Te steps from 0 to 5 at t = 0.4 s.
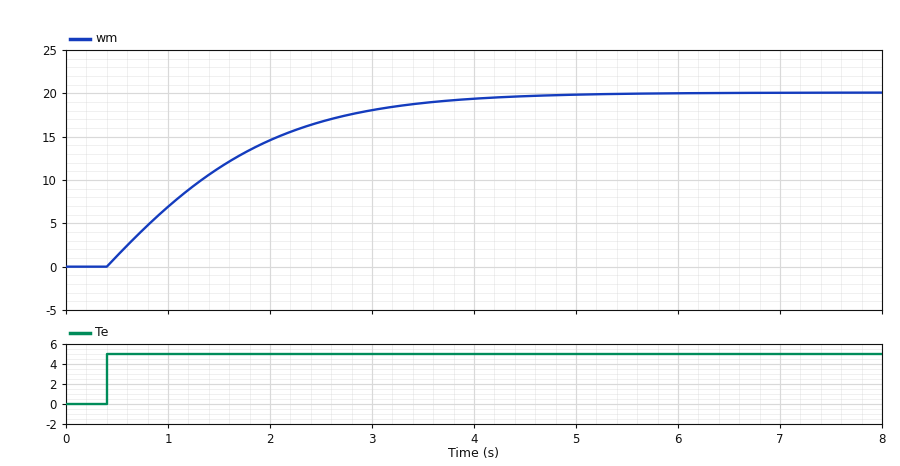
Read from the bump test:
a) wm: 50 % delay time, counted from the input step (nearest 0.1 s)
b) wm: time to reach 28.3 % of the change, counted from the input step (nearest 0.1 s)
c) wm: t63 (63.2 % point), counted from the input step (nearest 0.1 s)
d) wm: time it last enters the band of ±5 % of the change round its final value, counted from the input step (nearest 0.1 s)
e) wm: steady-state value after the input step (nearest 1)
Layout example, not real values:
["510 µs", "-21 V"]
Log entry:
["0.9 s", "0.5 s", "1.3 s", "3.3 s", "20"]
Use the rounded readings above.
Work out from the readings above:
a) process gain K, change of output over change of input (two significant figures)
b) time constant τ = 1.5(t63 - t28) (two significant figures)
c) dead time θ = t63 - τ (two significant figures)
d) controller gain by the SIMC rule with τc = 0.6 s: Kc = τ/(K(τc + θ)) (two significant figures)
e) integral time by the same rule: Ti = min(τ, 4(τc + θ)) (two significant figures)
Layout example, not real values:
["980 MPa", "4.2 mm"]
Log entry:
["4.0", "1.2 s", "0.10 s", "0.43", "1.2 s"]
